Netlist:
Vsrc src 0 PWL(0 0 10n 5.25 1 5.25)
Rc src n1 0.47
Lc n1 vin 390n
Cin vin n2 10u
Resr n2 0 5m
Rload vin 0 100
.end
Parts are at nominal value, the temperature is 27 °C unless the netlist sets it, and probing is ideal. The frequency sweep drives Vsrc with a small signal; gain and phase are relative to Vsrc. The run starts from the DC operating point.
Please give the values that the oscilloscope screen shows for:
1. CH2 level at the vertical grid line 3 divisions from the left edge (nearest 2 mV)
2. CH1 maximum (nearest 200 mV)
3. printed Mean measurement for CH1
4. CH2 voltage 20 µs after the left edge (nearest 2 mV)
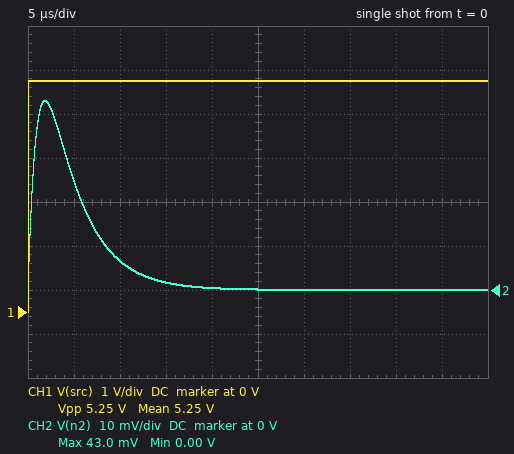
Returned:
2 mV
5.2 V
5.25 V
0 V
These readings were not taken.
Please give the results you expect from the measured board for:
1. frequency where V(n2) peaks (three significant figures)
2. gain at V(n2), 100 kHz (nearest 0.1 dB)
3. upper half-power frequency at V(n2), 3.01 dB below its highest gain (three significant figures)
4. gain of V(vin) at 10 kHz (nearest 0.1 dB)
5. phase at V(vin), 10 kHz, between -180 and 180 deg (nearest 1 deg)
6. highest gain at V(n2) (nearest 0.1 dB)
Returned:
80.8 kHz
-39.7 dB
223 kHz
-0.3 dB
-17 deg
-39.6 dB
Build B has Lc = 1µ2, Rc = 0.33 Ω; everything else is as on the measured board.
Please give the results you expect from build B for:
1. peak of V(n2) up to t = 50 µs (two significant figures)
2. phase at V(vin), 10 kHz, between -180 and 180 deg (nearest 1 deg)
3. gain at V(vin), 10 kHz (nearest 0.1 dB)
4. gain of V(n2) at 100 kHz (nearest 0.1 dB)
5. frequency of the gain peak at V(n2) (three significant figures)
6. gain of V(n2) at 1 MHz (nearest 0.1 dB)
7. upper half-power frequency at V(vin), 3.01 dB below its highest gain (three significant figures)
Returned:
42 mV
-12 deg
0.2 dB
-42.7 dB
46.0 kHz
-63.6 dB
54.0 kHz
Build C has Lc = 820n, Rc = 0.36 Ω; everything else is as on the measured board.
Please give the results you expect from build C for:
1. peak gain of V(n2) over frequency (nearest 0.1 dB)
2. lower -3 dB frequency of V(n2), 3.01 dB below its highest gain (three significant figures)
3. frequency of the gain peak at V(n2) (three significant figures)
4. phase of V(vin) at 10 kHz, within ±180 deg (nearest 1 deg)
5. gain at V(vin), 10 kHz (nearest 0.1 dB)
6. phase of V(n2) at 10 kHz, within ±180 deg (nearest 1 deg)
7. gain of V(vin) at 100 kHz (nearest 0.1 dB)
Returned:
-37.3 dB
30.5 kHz
55.7 kHz
-13 deg
0 dB
77 deg
-10.1 dB
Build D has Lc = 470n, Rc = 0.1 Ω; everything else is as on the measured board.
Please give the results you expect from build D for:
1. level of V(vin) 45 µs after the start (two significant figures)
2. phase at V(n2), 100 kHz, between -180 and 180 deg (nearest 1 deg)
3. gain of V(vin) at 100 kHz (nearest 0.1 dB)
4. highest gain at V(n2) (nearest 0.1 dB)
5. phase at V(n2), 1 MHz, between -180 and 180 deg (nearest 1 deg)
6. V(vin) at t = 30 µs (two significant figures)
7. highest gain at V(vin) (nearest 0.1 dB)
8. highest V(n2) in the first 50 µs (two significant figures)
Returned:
5.2 V
-52 deg
-0.7 dB
-26.5 dB
-88 deg
5.1 V
6.5 dB
87 mV
